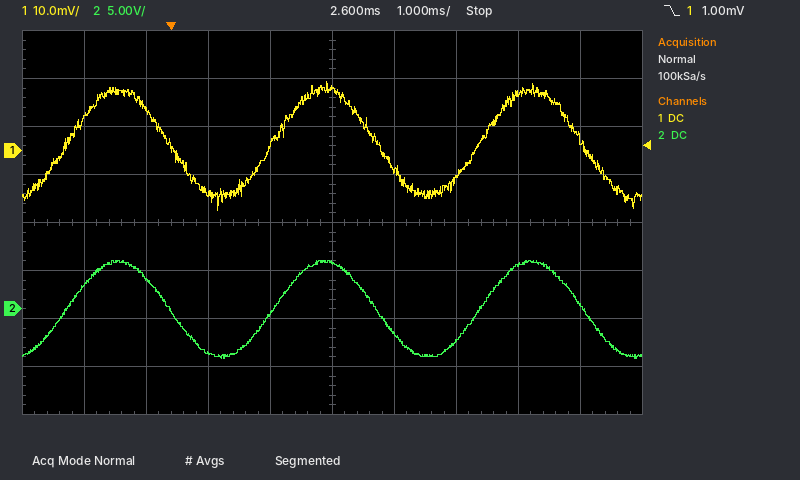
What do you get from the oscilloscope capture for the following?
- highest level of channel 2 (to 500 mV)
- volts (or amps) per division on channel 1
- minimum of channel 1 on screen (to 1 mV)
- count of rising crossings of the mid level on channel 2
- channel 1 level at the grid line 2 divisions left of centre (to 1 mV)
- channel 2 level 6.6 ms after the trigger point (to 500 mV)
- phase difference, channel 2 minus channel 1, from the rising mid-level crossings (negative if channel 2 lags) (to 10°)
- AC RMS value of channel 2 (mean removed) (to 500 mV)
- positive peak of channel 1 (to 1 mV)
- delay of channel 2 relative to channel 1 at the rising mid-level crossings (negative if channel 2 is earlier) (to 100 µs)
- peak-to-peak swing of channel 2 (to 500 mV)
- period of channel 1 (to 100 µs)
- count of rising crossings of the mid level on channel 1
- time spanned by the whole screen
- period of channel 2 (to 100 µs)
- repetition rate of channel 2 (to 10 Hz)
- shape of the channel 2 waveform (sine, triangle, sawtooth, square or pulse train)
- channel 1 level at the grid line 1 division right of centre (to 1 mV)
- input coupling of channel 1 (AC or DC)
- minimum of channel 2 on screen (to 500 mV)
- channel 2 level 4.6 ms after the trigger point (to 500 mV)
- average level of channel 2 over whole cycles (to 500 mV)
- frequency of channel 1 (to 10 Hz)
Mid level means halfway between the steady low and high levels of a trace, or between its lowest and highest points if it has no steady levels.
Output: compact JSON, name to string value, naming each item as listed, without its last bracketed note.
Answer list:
{"highest level of channel 2": "5.0 V", "volts (or amps) per division on channel 1": "10 mV", "minimum of channel 1 on screen": "-12 mV", "count of rising crossings of the mid level on channel 2": "3", "channel 1 level at the grid line 2 divisions left of centre": "-9 mV", "channel 2 level 6.6 ms after the trigger point": "500 mV", "phase difference, channel 2 minus channel 1, from the rising mid-level crossings (negative if channel 2 lags)": "0°", "AC RMS value of channel 2 (mean removed)": "3.5 V", "positive peak of channel 1": "14 mV", "delay of channel 2 relative to channel 1 at the rising mid-level crossings (negative if channel 2 is earlier)": "0.0 ms", "peak-to-peak swing of channel 2": "10.0 V", "period of channel 1": "3.3 ms", "count of rising crossings of the mid level on channel 1": "3", "time spanned by the whole screen": "10 ms", "period of channel 2": "3.3 ms", "repetition rate of channel 2": "300 Hz", "shape of the channel 2 waveform": "sine", "channel 1 level at the grid line 1 division right of centre": "-4 mV", "input coupling of channel 1": "DC", "minimum of channel 2 on screen": "-5.0 V", "channel 2 level 4.6 ms after the trigger point": "-3.5 V", "average level of channel 2 over whole cycles": "0.0 V", "frequency of channel 1": "300 Hz"}
